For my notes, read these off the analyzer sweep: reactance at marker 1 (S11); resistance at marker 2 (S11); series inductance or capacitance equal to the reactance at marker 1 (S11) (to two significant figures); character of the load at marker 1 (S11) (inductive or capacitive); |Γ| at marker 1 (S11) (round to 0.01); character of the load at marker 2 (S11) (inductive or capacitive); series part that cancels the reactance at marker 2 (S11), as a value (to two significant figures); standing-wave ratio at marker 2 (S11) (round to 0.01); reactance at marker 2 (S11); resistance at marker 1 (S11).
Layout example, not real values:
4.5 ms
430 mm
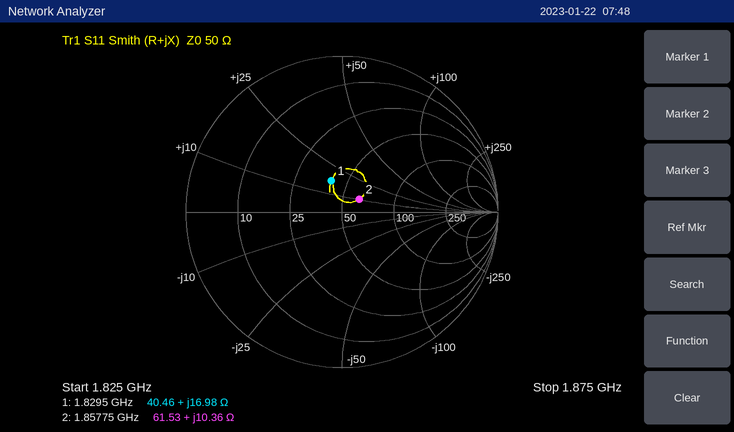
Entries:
+16.98 Ω
61.53 Ω
1.5 nH
inductive
0.21
inductive
8.3 pF
1.32
+10.36 Ω
40.46 Ω
